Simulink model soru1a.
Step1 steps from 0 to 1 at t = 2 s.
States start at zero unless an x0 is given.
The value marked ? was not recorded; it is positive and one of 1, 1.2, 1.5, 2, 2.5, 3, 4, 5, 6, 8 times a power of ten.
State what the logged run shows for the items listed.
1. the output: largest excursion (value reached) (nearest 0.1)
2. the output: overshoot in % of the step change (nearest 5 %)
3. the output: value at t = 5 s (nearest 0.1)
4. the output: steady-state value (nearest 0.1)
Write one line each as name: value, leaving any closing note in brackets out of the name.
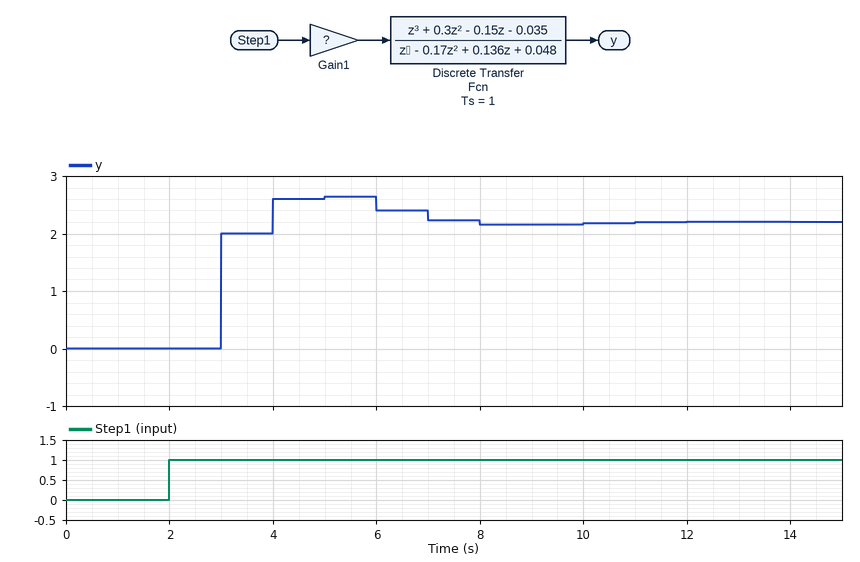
the output: largest excursion (value reached): 2.6
the output: overshoot in % of the step change: 20 %
the output: value at t = 5 s: 2.6
the output: steady-state value: 2.2
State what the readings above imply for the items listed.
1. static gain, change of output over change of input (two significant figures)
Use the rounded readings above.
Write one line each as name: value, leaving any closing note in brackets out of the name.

static gain, change of output over change of input: 2.2
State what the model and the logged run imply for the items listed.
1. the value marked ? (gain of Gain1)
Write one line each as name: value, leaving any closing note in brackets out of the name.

the value marked ?: 2
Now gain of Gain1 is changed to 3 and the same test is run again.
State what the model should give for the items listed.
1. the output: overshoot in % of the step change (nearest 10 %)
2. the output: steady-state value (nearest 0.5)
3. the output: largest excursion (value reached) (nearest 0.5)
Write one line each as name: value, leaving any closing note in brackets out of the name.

the output: overshoot in % of the step change: 20 %
the output: steady-state value: 3.5
the output: largest excursion (value reached): 4.0
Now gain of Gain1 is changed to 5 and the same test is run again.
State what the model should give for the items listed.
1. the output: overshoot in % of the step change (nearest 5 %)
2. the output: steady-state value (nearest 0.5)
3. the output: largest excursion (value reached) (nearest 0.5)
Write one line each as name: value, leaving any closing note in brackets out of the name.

the output: overshoot in % of the step change: 20 %
the output: steady-state value: 5.5
the output: largest excursion (value reached): 6.5
